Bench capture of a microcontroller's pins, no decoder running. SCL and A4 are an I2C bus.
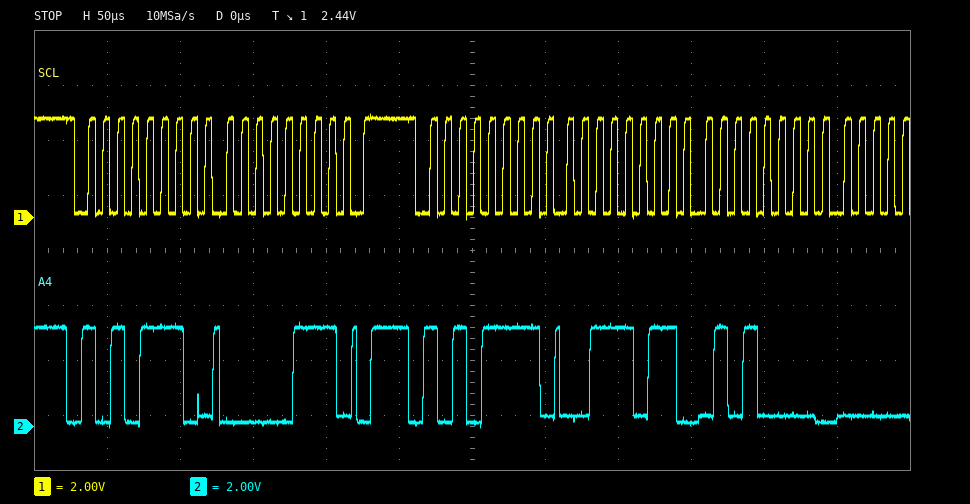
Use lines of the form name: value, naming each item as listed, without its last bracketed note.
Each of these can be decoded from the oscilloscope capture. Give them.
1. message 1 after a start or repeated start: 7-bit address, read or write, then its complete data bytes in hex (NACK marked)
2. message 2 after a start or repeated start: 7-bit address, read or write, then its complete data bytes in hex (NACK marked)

message 1 after a start or repeated start: 7-bit address, read or write, then its complete data bytes in hex: 0x57 write: 07
message 2 after a start or repeated start: 7-bit address, read or write, then its complete data bytes in hex: 0x57 read: 3B 50
